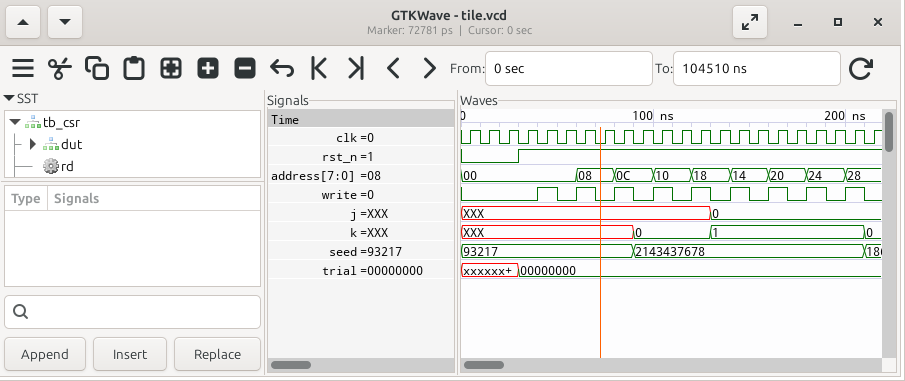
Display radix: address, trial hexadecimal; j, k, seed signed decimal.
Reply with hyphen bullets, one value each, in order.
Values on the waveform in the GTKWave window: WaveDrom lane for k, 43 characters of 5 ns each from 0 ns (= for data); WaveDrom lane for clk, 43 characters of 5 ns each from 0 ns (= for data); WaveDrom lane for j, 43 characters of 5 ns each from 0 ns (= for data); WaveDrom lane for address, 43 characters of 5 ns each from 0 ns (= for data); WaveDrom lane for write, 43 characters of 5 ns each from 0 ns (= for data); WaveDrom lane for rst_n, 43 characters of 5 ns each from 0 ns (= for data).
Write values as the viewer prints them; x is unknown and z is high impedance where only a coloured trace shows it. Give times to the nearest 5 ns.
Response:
- {name: 'k', wave: 'x.................=.......=...............=', data: '0 1 0'}
- {name: 'clk', wave: '0101010101010101010101010101010101010101010'}
- {name: 'j', wave: 'x.........................=................', data: '0'}
- {name: 'address', wave: '=...........=...=...=...=...=...=...=...=..', data: '00 08 0C 10 18 14 20 24 28'}
- {name: 'write', wave: '0.......1.0.1.0.1.0.1.0.1.0.1.0.1.0.1.0.1.0'}
- {name: 'rst_n', wave: '0.....1....................................'}
